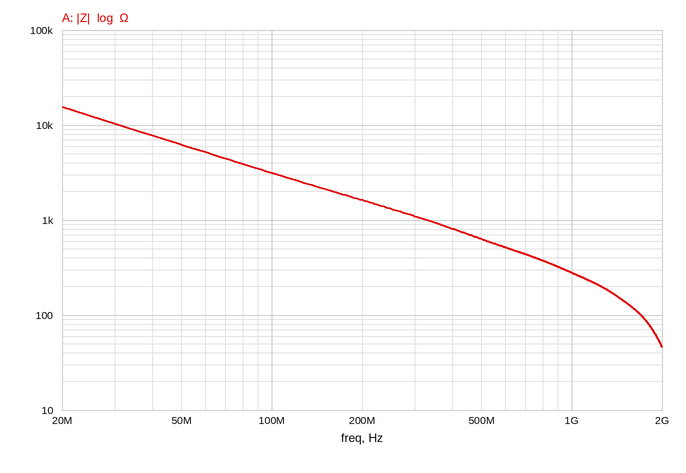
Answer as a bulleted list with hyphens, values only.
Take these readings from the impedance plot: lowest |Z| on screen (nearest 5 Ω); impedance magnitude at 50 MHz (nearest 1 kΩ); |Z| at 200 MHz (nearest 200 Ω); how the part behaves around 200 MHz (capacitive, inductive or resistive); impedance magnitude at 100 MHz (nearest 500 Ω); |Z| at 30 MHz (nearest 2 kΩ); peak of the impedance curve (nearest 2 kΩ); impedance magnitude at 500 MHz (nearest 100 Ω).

- 45 Ω
- 6 kΩ
- 1.6 kΩ
- capacitive
- 3.0 kΩ
- 10 kΩ
- 16 kΩ
- 600 Ω
